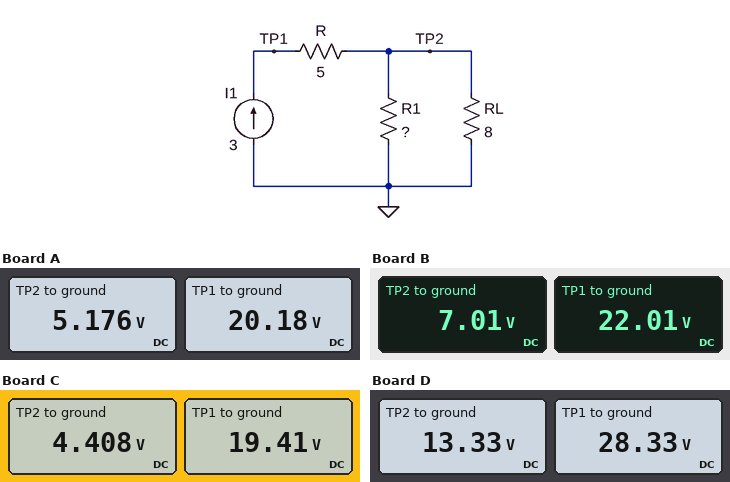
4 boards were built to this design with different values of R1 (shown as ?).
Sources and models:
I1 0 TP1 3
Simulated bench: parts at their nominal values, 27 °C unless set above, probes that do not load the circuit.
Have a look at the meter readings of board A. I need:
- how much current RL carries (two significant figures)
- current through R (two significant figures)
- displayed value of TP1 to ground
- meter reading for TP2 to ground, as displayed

650 mA
3.0 A
20.18 V
5.176 V
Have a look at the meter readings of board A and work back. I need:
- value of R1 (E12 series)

2.2 Ω
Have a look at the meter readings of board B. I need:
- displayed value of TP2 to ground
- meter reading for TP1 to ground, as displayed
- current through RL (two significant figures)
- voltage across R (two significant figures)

7.01 V
22.01 V
880 mA
15 V
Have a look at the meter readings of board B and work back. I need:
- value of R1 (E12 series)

3.3 Ω
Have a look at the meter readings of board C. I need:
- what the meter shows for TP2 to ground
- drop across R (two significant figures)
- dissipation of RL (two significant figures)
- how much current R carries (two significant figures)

4.408 V
15 V
2.4 W
3.0 A
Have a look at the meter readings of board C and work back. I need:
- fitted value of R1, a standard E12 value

1.8 Ω
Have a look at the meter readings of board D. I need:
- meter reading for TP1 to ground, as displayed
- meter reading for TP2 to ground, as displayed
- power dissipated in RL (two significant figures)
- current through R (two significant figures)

28.33 V
13.33 V
22 W
3.0 A
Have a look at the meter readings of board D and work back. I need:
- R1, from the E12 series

10 Ω
